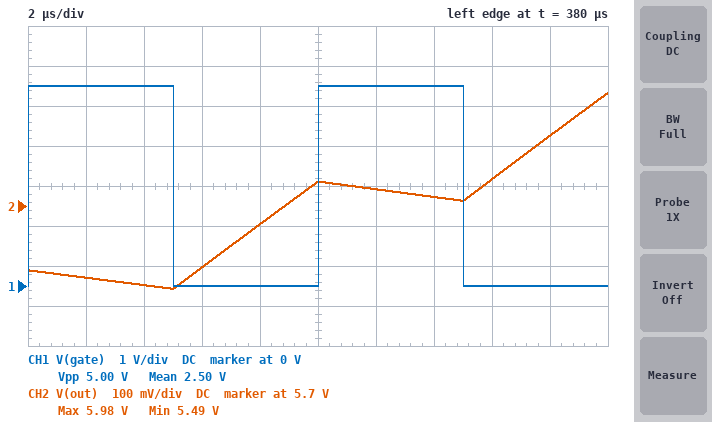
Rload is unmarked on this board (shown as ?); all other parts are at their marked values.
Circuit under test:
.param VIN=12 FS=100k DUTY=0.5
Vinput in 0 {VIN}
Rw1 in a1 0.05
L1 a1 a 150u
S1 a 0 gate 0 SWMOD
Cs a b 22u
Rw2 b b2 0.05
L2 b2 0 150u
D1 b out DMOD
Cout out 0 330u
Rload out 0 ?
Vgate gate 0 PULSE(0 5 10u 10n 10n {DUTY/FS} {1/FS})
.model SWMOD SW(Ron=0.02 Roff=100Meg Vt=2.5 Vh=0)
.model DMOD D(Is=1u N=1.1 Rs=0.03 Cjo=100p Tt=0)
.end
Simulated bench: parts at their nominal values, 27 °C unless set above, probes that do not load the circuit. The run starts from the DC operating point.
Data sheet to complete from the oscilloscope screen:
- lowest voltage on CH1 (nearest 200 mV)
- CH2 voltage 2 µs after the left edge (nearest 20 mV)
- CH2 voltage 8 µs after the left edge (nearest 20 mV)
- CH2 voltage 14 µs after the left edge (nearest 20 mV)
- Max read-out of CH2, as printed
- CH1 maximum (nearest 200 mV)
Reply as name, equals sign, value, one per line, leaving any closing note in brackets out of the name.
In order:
lowest voltage on CH1 = 0 V
CH2 voltage 2 µs after the left edge = 5.52 V
CH2 voltage 8 µs after the left edge = 5.66 V
CH2 voltage 14 µs after the left edge = 5.72 V
Max read-out of CH2, as printed = 5.98 V
CH1 maximum = 5.0 V
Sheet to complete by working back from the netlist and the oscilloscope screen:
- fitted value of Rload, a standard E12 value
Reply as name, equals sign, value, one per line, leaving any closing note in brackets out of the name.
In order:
fitted value of Rload, a standard E12 value = 1.8 Ω
